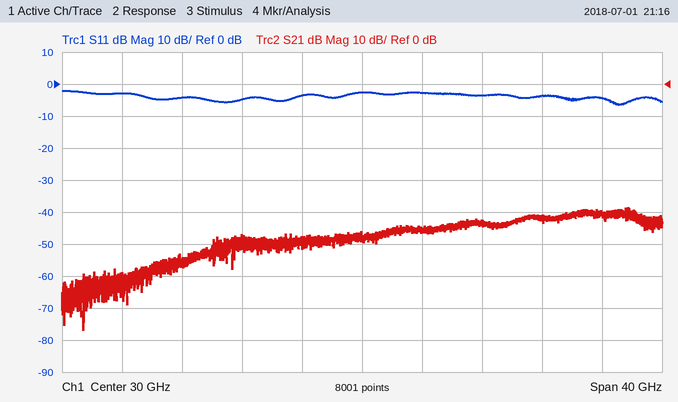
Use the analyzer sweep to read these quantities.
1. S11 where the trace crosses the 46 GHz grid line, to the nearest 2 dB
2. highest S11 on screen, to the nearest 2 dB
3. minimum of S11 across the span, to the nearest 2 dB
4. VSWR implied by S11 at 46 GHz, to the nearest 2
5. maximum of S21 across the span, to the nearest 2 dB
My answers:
-4 dB
-2 dB
-6 dB
4
-38 dB
